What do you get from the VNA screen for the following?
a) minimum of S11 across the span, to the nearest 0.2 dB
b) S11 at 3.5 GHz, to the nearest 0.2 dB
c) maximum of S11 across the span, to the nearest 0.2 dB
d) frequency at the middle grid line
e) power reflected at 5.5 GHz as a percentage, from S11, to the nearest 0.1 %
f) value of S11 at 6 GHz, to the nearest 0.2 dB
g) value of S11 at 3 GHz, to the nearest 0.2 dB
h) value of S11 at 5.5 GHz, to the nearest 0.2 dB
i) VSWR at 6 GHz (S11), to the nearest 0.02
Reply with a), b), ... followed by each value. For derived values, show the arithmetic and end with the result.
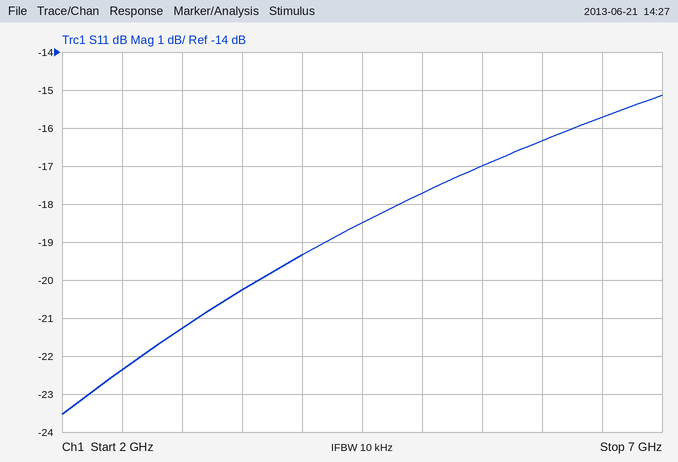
a) -23.6 dB
b) -20.2 dB
c) -15.2 dB
d) 4.5 GHz
e) 10^(-17/10) ≈ 2.0 %
f) -16.4 dB
g) -21.2 dB
h) -17.0 dB
i) |Γ| = 10^(-16.4/20) = 0.1514; VSWR = (1 + 0.1514)/(1 − 0.1514) ≈ 1.36
